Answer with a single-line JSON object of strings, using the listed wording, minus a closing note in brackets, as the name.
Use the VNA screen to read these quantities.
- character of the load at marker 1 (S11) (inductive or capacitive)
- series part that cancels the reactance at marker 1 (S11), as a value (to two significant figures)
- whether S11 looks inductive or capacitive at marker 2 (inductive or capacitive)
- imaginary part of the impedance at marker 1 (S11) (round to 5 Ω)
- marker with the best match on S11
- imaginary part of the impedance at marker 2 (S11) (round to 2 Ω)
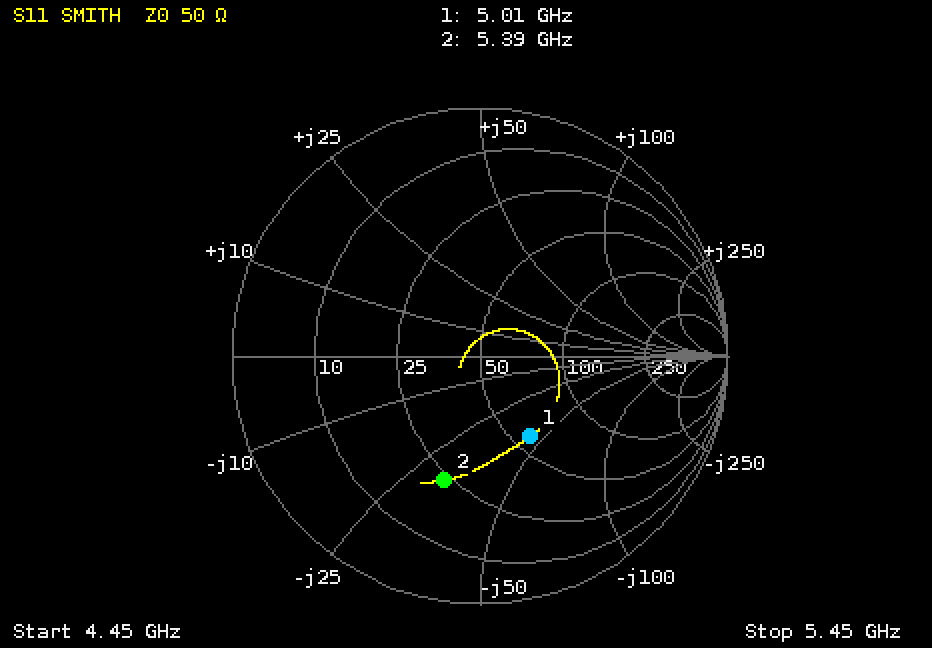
{"character of the load at marker 1 (S11)": "capacitive", "series part that cancels the reactance at marker 1 (S11), as a value": "1.4 nH", "whether S11 looks inductive or capacitive at marker 2": "capacitive", "imaginary part of the impedance at marker 1 (S11)": "-45 Ω", "marker with the best match on S11": "marker 1", "imaginary part of the impedance at marker 2 (S11)": "-32 Ω"}
